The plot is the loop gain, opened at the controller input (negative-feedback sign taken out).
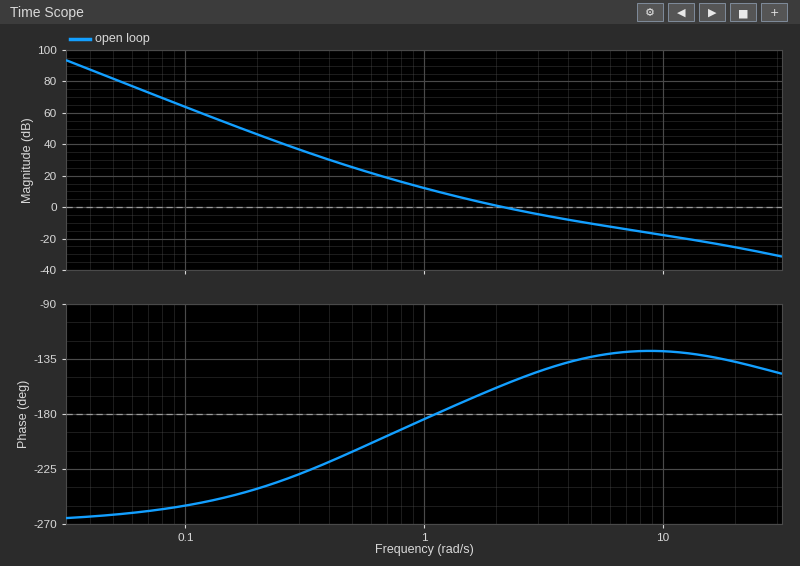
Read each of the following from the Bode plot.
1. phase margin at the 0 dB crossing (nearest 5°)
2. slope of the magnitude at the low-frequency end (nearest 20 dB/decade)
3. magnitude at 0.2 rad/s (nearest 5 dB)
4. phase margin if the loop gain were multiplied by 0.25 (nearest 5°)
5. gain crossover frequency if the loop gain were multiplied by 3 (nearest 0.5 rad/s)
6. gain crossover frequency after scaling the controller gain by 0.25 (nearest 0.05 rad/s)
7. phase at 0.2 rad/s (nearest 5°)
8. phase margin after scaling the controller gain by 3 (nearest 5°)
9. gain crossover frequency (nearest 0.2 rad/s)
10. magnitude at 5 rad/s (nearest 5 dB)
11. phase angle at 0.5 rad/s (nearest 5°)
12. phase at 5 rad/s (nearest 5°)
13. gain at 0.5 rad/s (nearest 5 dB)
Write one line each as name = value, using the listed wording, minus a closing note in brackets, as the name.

phase margin at the 0 dB crossing = 25°
slope of the magnitude at the low-frequency end = -60 dB/decade
magnitude at 0.2 rad/s = 45 dB
phase margin if the loop gain were multiplied by 0.25 = -5°
gain crossover frequency if the loop gain were multiplied by 3 = 4.5 rad/s
gain crossover frequency after scaling the controller gain by 0.25 = 1.00 rad/s
phase at 0.2 rad/s = -240°
phase margin after scaling the controller gain by 3 = 45°
gain crossover frequency = 2.2 rad/s
magnitude at 5 rad/s = -10 dB
phase angle at 0.5 rad/s = -210°
phase at 5 rad/s = -135°
gain at 0.5 rad/s = 25 dB
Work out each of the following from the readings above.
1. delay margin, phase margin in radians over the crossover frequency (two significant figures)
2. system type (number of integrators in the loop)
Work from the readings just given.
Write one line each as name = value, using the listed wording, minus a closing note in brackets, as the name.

delay margin, phase margin in radians over the crossover frequency = 0.20 s
system type = 3
